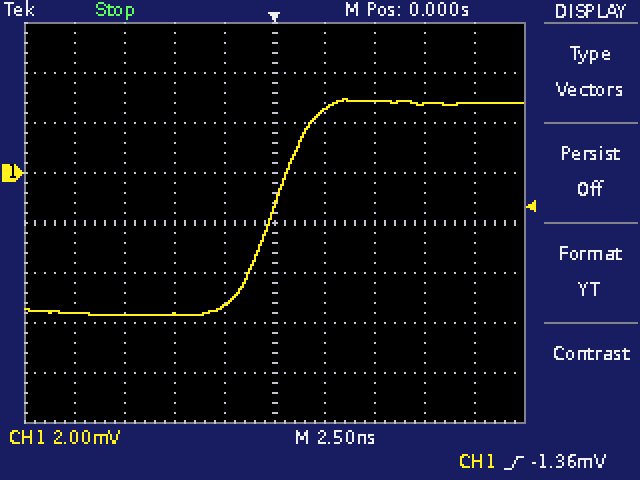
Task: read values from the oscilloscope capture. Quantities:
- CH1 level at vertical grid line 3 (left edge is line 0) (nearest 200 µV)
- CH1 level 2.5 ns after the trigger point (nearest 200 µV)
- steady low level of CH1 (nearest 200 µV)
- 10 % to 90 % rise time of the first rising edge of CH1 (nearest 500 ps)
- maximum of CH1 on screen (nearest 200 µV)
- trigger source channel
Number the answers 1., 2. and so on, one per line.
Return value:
1. -5.6 mV
2. 2.6 mV
3. -5.6 mV
4. 3.5 ns
5. 3.0 mV
6. CH1
